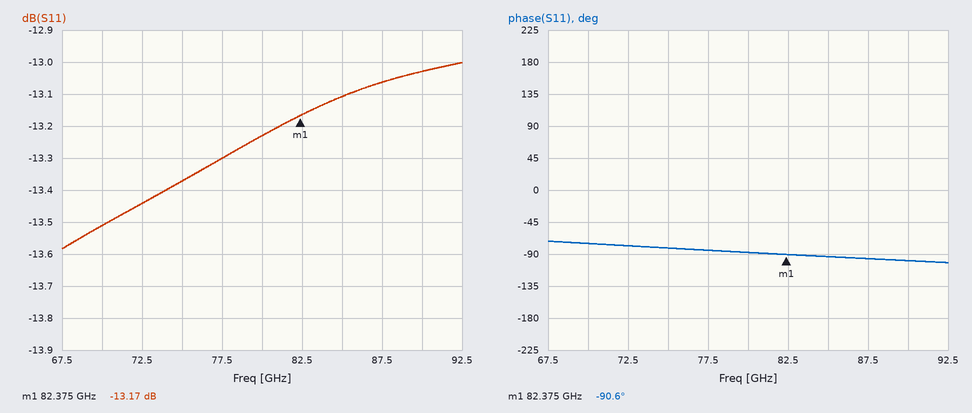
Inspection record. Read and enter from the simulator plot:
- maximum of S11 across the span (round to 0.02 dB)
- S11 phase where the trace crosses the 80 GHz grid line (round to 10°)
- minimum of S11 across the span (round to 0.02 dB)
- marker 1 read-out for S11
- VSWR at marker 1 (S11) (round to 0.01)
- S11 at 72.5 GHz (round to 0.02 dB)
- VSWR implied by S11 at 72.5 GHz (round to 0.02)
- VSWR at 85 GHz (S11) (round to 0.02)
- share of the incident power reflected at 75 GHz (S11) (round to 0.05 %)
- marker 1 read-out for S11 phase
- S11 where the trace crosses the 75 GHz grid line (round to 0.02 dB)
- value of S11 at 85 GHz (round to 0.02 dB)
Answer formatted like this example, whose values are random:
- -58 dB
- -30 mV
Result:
- -13.00 dB
- -90°
- -13.58 dB
- -13.17 dB
- 1.56
- -13.44 dB
- 1.54
- 1.56
- 4.60 %
- -90.6°
- -13.38 dB
- -13.10 dB
